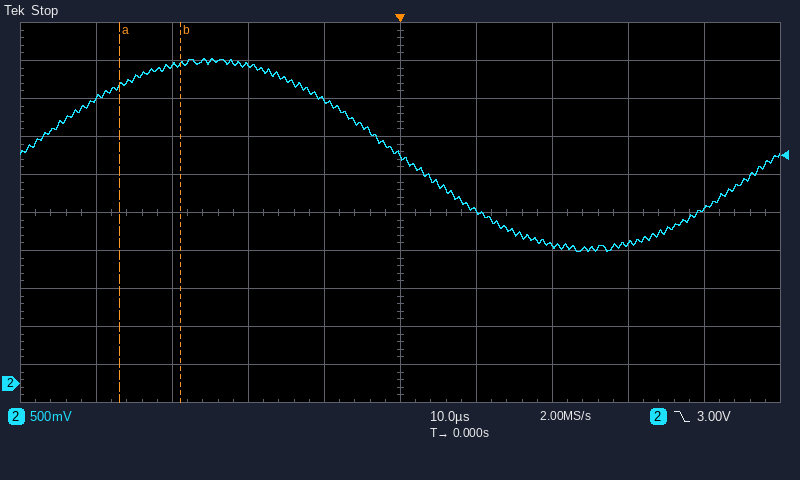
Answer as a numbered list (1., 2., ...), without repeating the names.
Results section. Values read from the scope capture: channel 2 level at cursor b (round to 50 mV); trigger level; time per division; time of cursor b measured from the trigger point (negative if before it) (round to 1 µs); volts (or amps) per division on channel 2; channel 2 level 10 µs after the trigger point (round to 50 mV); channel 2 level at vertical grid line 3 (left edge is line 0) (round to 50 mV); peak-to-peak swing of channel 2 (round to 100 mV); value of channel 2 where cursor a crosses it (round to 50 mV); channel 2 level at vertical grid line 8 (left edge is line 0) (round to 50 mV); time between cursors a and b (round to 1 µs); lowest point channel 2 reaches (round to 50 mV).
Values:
1. 4.20 V
2. 3.00 V
3. 10 µs
4. -29 µs
5. 500 mV
6. 2.25 V
7. 4.20 V
8. 2.50 V
9. 3.90 V
10. 1.85 V
11. 8 µs
12. 1.75 V
